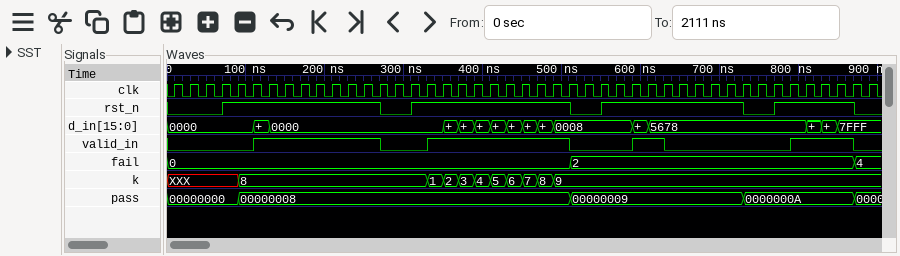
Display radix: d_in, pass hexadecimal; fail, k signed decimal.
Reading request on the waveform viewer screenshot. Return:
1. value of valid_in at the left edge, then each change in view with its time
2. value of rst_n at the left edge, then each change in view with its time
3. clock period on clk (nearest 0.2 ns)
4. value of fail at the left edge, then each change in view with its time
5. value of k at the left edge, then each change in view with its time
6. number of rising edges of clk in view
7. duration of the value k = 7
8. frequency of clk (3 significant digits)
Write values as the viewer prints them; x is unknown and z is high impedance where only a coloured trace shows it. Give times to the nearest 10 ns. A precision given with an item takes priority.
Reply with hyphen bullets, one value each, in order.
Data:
- 0, 1 at 110 ns, 0 at 270 ns, 1 at 330 ns, 0 at 510 ns, 1 at 590 ns, 0 at 630 ns, 1 at 790 ns, 0 at 870 ns
- 0, 1 at 70 ns, 0 at 270 ns, 1 at 310 ns, 0 at 510 ns, 1 at 550 ns, 0 at 730 ns, 1 at 770 ns, 0 at 870 ns
- 20 ns
- 0, 2 at 510 ns, 4 at 870 ns
- XXX, 8 at 90 ns, 1 at 330 ns, 2 at 350 ns, 3 at 370 ns, 4 at 390 ns, 5 at 410 ns, 6 at 430 ns, 7 at 450 ns, 8 at 470 ns, 9 at 490 ns
- 45
- 20 ns
- 50.0 MHz
